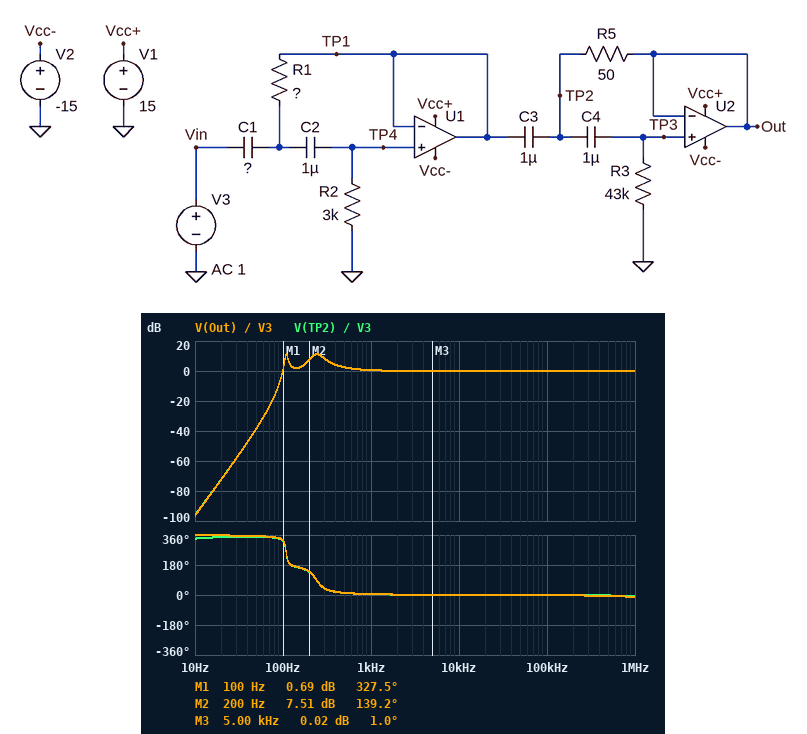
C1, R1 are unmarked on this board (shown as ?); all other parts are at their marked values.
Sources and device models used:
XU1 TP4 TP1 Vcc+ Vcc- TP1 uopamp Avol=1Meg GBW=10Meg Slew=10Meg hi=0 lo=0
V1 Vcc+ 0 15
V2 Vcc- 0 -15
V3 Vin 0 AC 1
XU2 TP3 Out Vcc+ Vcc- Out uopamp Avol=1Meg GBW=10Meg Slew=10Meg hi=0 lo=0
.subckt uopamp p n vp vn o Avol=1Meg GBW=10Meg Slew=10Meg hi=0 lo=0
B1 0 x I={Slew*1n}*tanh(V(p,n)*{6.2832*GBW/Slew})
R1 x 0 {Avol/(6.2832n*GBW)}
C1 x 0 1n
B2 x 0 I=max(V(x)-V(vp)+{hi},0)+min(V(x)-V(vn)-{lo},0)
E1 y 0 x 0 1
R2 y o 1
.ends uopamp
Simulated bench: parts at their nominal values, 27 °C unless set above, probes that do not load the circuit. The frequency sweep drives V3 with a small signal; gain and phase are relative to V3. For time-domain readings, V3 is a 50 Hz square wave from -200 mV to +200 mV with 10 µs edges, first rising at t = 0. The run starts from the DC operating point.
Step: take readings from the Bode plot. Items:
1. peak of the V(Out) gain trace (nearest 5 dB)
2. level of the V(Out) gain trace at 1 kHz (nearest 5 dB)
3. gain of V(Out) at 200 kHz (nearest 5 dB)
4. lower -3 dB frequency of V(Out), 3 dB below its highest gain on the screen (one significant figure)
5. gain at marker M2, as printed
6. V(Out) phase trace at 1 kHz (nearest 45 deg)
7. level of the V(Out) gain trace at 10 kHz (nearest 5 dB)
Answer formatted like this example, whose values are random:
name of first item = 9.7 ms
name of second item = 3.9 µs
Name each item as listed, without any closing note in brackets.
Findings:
peak of the V(Out) gain trace = 10 dB
level of the V(Out) gain trace at 1 kHz = 0 dB
gain of V(Out) at 200 kHz = 0 dB
lower -3 dB frequency of V(Out), 3 dB below its highest gain on the screen = 100 Hz
gain at marker M2, as printed = 7.51 dB
V(Out) phase trace at 1 kHz = 0 deg
level of the V(Out) gain trace at 10 kHz = 0 dB
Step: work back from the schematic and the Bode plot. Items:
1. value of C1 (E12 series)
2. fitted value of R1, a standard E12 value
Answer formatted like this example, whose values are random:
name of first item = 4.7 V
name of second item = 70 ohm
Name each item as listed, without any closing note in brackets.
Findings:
value of C1 = 1.8 µF
fitted value of R1, a standard E12 value = 82 Ω
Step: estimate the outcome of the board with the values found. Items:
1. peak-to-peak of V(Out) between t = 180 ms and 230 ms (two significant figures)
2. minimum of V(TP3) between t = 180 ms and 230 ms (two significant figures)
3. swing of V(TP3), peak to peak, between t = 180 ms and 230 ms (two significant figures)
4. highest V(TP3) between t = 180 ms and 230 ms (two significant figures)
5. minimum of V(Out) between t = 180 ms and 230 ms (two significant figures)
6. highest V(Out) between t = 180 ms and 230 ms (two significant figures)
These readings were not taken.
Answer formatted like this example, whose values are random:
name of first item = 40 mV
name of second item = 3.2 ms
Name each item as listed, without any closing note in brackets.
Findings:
peak-to-peak of V(Out) between t = 180 ms and 230 ms = 940 mV
minimum of V(TP3) between t = 180 ms and 230 ms = -470 mV
swing of V(TP3), peak to peak, between t = 180 ms and 230 ms = 940 mV
highest V(TP3) between t = 180 ms and 230 ms = 470 mV
minimum of V(Out) between t = 180 ms and 230 ms = -470 mV
highest V(Out) between t = 180 ms and 230 ms = 470 mV
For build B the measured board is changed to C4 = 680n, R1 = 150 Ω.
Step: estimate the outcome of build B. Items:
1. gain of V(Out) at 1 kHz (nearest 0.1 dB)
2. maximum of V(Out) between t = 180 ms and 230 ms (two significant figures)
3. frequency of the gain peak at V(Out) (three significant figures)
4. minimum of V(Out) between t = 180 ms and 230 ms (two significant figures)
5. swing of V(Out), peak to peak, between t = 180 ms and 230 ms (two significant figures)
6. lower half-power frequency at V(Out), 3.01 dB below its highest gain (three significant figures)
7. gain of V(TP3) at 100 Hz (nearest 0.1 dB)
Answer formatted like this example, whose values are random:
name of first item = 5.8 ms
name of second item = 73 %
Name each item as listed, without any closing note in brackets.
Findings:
gain of V(Out) at 1 kHz = 0.4 dB
maximum of V(Out) between t = 180 ms and 230 ms = 660 mV
frequency of the gain peak at V(Out) = 132 Hz
minimum of V(Out) between t = 180 ms and 230 ms = -660 mV
swing of V(Out), peak to peak, between t = 180 ms and 230 ms = 1.3 V
lower half-power frequency at V(Out), 3.01 dB below its highest gain = 128 Hz
gain of V(TP3) at 100 Hz = -4.5 dB
